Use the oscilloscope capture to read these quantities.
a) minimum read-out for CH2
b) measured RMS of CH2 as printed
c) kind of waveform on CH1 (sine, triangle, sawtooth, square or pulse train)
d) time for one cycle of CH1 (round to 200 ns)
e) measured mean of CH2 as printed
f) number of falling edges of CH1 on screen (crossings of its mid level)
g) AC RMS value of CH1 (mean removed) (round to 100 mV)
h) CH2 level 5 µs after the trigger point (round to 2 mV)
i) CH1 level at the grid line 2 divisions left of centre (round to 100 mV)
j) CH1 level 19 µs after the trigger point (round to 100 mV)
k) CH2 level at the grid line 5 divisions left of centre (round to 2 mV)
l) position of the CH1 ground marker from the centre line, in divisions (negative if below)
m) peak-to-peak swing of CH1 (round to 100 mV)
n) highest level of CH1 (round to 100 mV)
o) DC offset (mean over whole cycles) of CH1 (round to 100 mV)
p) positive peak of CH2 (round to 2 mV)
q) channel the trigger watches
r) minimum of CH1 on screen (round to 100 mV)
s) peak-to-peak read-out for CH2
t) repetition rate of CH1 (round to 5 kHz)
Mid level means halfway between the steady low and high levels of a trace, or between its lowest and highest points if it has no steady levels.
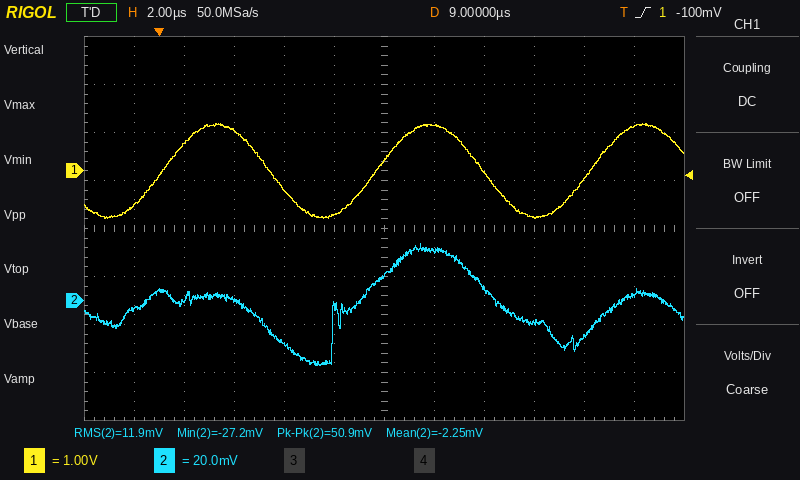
-27.2 mV
11.9 mV
sine
8.6 µs
-2.25 mV
2
700 mV
-18 mV
-400 mV
900 mV
-4 mV
+1.2 div
2.0 V
1.0 V
0.0 V
24 mV
CH1
-1.0 V
50.9 mV
115 kHz
